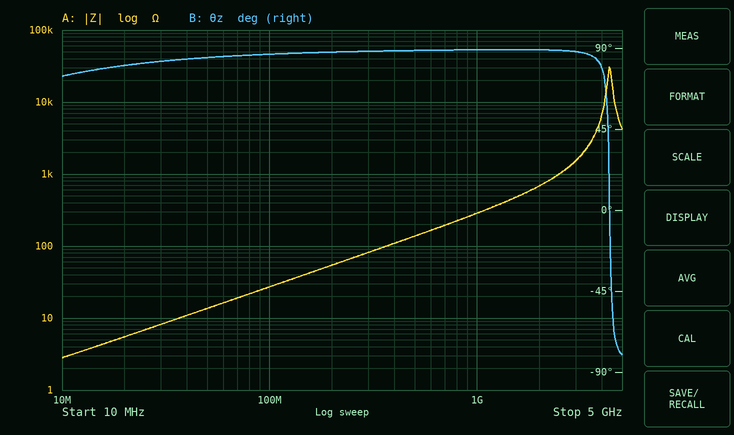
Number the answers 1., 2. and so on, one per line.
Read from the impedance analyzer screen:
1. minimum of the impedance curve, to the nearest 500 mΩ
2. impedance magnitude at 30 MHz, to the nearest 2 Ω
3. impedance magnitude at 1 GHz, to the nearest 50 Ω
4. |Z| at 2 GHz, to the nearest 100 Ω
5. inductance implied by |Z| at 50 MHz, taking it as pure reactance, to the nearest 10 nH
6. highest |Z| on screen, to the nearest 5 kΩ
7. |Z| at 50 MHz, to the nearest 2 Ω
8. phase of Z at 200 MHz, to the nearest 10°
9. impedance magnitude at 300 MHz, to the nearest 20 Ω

1. 3.0 Ω
2. 8 Ω
3. 300 Ω
4. 700 Ω
5. 40 nH
6. 30 kΩ
7. 14 Ω
8. 90°
9. 80 Ω
